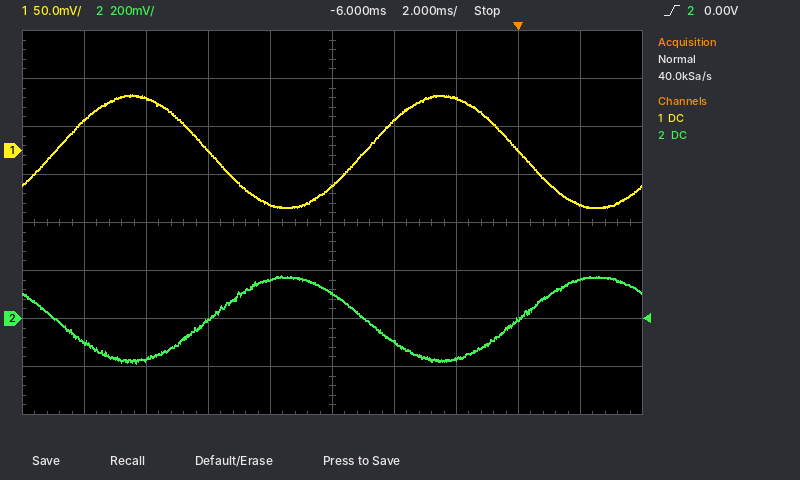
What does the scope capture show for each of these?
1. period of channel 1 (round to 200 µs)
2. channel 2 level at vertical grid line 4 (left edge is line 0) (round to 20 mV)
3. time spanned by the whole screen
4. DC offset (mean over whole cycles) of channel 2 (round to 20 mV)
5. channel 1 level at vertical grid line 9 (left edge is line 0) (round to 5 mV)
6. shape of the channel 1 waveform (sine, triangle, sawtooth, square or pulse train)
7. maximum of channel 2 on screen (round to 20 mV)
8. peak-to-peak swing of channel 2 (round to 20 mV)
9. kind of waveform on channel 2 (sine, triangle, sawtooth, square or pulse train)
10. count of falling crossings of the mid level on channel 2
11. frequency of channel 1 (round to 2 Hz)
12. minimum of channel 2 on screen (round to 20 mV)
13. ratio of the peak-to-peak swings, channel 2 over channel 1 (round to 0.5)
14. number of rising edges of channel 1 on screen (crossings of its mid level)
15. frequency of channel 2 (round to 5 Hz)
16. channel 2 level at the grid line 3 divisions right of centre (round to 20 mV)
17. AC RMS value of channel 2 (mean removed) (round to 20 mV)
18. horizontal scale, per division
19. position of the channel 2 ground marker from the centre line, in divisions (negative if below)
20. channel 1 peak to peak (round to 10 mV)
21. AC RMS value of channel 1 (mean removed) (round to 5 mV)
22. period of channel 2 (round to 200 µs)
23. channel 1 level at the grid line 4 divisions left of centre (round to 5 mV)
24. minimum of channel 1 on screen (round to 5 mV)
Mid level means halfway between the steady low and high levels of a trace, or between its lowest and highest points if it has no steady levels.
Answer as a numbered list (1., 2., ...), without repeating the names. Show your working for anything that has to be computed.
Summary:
1. 10.0 ms
2. 160 mV
3. 20 ms
4. (180 mV + (-180 mV)) / 2 ≈ 0 mV
5. -55 mV
6. sine
7. 180 mV
8. 180 mV − (-180 mV) = 360 mV
9. sine
10. 2
11. 1 / 10.0 ms ≈ 100 Hz
12. -180 mV
13. 360 mV / 120 mV ≈ 3.0
14. 2
15. 1 / 10.0 ms ≈ 100 Hz
16. 0 mV
17. 360 mV / (2√2) ≈ 127 mV, so 120 mV to the nearest 20 mV
18. 2 ms
19. -2.0 div
20. 120 mV
21. 120 mV / (2√2) ≈ 42.4 mV, so 40 mV to the nearest 5 mV
22. 10.0 ms
23. 30 mV
24. -60 mV
